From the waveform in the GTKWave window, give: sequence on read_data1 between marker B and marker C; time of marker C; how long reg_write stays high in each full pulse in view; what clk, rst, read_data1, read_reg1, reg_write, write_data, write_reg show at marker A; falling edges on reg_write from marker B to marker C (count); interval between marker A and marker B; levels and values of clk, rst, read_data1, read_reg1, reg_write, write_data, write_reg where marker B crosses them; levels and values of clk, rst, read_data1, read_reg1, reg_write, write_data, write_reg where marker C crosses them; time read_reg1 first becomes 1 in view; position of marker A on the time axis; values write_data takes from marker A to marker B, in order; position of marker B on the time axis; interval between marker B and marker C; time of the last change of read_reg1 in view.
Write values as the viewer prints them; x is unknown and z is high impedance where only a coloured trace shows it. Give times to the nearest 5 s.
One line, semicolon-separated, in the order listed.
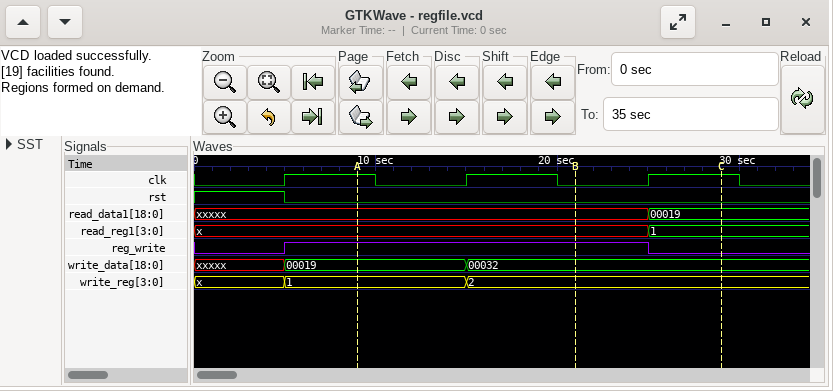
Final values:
xxxxx, 00019; 30 s; 20 s; clk=1, rst=0, read_data1=xxxxx, read_reg1=x, reg_write=1, write_data=00019, write_reg=1; 1; 10 s; clk=0, rst=0, read_data1=xxxxx, read_reg1=x, reg_write=1, write_data=00032, write_reg=2; clk=1, rst=0, read_data1=00019, read_reg1=1, reg_write=0, write_data=00032, write_reg=2; 25 s; 10 s; 00019, 00032; 20 s; 10 s; 25 s
